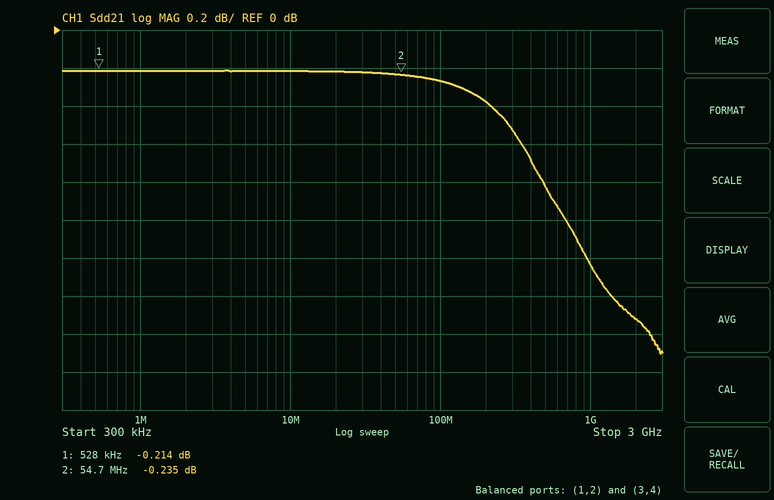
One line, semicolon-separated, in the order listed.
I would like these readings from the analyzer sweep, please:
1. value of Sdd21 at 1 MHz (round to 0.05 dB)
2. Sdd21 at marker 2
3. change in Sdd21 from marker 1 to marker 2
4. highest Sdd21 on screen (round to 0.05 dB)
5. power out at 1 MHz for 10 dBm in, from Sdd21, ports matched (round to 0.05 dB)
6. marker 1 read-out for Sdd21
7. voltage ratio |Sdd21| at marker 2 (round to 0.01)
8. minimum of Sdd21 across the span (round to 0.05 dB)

-0.20 dB; -0.235 dB; -0.021 dB; -0.20 dB; 9.80 dBm; -0.214 dB; 0.97; -1.70 dB
